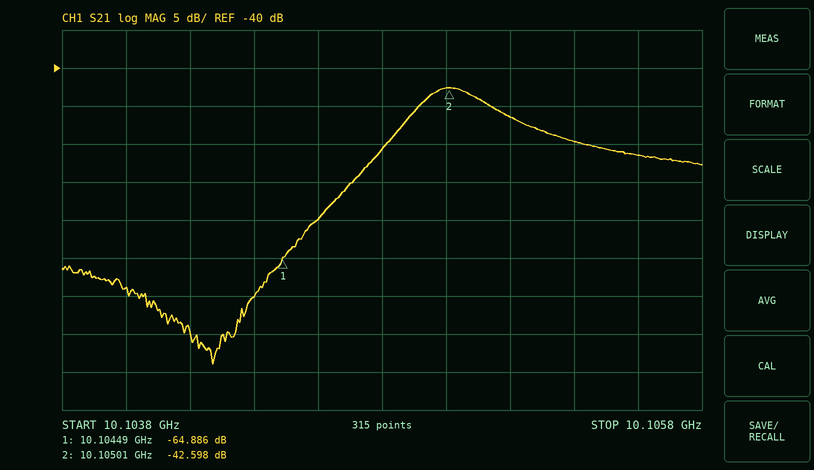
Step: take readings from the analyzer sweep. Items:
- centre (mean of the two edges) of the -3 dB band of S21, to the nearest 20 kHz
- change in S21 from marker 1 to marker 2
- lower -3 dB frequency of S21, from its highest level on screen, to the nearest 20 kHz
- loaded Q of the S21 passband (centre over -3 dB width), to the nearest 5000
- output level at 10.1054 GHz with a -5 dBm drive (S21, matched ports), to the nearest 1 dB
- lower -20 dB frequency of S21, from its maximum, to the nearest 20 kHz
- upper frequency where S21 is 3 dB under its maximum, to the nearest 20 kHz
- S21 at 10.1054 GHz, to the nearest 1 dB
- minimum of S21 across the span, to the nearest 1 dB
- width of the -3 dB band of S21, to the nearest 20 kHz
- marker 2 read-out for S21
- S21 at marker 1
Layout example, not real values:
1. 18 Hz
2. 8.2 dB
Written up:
1. 10.10504 GHz
2. 22.288 dB
3. 10.10490 GHz
4. 40000
5. -55 dBm
6. 10.10454 GHz
7. 10.10516 GHz
8. -50 dB
9. -79 dB
10. 260 kHz
11. -42.598 dB
12. -64.886 dB
